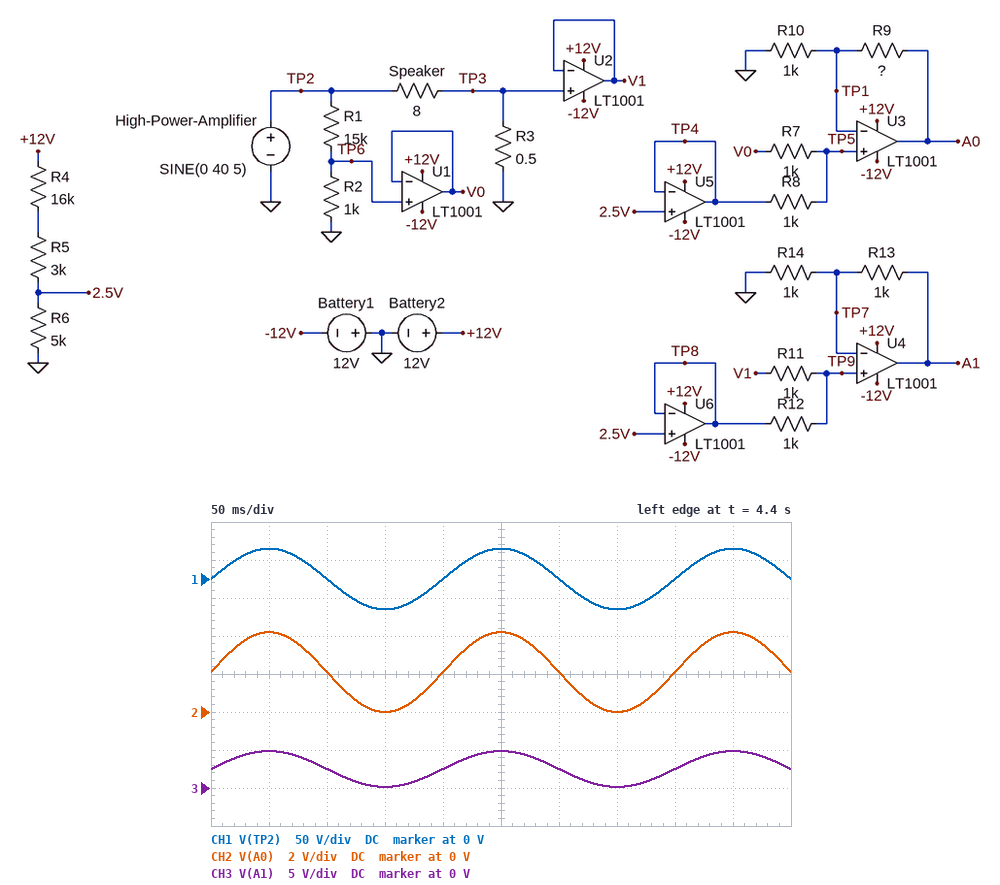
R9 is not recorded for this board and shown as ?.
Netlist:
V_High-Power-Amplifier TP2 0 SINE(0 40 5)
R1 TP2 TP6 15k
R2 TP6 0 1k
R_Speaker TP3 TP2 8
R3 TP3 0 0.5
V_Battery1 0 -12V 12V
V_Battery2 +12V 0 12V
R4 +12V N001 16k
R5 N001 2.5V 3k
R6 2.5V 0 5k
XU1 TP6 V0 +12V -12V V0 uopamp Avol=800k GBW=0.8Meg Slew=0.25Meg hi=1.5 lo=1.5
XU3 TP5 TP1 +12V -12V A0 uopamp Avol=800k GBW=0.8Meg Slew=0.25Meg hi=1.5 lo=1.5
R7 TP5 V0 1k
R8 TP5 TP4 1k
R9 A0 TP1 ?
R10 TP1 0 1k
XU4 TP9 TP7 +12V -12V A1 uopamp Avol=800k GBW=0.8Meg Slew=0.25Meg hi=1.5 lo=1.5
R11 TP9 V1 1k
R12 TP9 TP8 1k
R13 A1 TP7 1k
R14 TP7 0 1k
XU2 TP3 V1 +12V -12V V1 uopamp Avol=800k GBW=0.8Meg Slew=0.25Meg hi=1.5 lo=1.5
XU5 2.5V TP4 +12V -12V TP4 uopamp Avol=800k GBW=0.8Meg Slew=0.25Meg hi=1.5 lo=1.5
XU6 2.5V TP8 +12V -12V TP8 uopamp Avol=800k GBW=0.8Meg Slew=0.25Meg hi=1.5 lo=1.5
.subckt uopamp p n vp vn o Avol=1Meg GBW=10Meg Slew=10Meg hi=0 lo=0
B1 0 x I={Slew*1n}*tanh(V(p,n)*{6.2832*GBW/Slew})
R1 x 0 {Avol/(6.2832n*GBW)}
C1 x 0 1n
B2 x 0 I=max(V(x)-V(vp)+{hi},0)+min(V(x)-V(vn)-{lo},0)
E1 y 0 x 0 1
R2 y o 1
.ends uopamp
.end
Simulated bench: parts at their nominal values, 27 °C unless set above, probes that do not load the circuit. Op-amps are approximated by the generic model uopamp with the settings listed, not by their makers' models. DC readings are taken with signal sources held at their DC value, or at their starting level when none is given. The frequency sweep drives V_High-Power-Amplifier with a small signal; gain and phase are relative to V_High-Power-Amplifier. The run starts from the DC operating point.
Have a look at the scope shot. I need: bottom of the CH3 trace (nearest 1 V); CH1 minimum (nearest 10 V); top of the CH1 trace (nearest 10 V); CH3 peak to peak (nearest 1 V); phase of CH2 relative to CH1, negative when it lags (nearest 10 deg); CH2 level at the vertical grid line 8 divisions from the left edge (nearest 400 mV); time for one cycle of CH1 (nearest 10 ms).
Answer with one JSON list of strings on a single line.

["0 V", "-40 V", "40 V", "5 V", "0 deg", "2.0 V", "200 ms"]
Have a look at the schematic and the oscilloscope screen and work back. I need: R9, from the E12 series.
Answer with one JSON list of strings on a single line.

["680 Ω"]
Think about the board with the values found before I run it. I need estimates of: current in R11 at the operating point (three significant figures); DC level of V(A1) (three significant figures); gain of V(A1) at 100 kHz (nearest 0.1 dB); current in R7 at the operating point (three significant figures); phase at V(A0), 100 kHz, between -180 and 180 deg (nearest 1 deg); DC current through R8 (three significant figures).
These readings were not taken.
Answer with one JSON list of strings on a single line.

["1.25 mA", "2.50 V", "-24.9 dB", "1.25 mA", "-19 deg", "1.25 mA"]
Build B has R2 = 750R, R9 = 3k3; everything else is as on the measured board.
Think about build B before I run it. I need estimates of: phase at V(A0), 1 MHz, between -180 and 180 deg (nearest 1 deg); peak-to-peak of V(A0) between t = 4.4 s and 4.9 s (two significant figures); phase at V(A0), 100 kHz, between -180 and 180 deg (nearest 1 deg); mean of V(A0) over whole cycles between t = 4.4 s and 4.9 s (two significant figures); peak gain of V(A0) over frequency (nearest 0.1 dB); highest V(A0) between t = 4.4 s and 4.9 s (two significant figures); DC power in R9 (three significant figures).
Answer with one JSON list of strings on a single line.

["-131 deg", "8.2 V", "-35 deg", "5.4 V", "-19.8 dB", "9.5 V", "5.16 mW"]
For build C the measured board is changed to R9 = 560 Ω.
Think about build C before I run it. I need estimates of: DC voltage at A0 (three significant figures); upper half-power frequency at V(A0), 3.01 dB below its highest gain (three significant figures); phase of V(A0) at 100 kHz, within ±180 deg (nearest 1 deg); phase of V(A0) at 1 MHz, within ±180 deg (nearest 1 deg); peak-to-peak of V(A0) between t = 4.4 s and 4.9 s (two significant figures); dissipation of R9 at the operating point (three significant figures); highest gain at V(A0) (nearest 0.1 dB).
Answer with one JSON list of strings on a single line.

["1.95 V", "398 kHz", "-18 deg", "-114 deg", "3.9 V", "875 µW", "-26.2 dB"]
